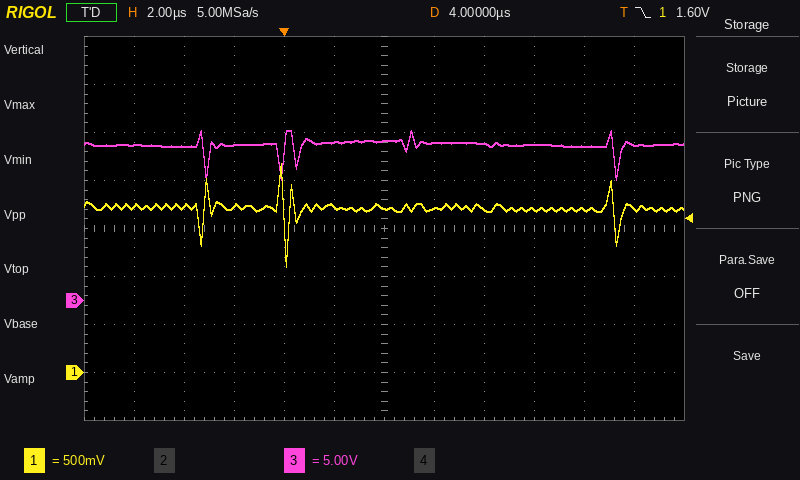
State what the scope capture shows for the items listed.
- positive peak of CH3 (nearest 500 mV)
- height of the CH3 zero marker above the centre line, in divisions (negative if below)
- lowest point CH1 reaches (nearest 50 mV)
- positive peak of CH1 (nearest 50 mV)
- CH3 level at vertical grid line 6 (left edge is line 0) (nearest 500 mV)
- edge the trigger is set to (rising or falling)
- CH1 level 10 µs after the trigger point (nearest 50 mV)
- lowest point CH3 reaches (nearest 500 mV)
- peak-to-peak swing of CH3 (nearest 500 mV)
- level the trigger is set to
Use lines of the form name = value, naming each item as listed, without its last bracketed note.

positive peak of CH3 = 17.5 V
height of the CH3 zero marker above the centre line, in divisions = -1.5 div
lowest point CH1 reaches = 1.10 V
positive peak of CH1 = 2.20 V
CH3 level at vertical grid line 6 (left edge is line 0) = 16.5 V
edge the trigger is set to = falling
CH1 level 10 µs after the trigger point = 1.70 V
lowest point CH3 reaches = 12.5 V
peak-to-peak swing of CH3 = 5.0 V
level the trigger is set to = 1.60 V
